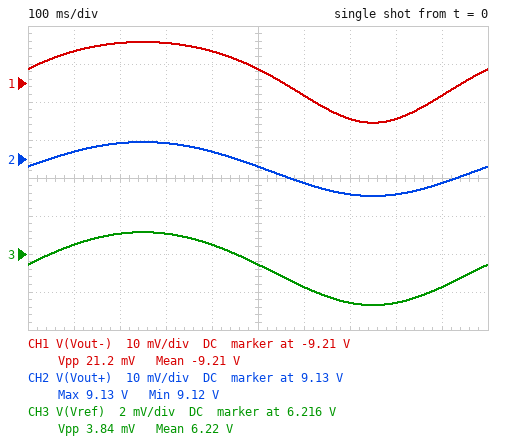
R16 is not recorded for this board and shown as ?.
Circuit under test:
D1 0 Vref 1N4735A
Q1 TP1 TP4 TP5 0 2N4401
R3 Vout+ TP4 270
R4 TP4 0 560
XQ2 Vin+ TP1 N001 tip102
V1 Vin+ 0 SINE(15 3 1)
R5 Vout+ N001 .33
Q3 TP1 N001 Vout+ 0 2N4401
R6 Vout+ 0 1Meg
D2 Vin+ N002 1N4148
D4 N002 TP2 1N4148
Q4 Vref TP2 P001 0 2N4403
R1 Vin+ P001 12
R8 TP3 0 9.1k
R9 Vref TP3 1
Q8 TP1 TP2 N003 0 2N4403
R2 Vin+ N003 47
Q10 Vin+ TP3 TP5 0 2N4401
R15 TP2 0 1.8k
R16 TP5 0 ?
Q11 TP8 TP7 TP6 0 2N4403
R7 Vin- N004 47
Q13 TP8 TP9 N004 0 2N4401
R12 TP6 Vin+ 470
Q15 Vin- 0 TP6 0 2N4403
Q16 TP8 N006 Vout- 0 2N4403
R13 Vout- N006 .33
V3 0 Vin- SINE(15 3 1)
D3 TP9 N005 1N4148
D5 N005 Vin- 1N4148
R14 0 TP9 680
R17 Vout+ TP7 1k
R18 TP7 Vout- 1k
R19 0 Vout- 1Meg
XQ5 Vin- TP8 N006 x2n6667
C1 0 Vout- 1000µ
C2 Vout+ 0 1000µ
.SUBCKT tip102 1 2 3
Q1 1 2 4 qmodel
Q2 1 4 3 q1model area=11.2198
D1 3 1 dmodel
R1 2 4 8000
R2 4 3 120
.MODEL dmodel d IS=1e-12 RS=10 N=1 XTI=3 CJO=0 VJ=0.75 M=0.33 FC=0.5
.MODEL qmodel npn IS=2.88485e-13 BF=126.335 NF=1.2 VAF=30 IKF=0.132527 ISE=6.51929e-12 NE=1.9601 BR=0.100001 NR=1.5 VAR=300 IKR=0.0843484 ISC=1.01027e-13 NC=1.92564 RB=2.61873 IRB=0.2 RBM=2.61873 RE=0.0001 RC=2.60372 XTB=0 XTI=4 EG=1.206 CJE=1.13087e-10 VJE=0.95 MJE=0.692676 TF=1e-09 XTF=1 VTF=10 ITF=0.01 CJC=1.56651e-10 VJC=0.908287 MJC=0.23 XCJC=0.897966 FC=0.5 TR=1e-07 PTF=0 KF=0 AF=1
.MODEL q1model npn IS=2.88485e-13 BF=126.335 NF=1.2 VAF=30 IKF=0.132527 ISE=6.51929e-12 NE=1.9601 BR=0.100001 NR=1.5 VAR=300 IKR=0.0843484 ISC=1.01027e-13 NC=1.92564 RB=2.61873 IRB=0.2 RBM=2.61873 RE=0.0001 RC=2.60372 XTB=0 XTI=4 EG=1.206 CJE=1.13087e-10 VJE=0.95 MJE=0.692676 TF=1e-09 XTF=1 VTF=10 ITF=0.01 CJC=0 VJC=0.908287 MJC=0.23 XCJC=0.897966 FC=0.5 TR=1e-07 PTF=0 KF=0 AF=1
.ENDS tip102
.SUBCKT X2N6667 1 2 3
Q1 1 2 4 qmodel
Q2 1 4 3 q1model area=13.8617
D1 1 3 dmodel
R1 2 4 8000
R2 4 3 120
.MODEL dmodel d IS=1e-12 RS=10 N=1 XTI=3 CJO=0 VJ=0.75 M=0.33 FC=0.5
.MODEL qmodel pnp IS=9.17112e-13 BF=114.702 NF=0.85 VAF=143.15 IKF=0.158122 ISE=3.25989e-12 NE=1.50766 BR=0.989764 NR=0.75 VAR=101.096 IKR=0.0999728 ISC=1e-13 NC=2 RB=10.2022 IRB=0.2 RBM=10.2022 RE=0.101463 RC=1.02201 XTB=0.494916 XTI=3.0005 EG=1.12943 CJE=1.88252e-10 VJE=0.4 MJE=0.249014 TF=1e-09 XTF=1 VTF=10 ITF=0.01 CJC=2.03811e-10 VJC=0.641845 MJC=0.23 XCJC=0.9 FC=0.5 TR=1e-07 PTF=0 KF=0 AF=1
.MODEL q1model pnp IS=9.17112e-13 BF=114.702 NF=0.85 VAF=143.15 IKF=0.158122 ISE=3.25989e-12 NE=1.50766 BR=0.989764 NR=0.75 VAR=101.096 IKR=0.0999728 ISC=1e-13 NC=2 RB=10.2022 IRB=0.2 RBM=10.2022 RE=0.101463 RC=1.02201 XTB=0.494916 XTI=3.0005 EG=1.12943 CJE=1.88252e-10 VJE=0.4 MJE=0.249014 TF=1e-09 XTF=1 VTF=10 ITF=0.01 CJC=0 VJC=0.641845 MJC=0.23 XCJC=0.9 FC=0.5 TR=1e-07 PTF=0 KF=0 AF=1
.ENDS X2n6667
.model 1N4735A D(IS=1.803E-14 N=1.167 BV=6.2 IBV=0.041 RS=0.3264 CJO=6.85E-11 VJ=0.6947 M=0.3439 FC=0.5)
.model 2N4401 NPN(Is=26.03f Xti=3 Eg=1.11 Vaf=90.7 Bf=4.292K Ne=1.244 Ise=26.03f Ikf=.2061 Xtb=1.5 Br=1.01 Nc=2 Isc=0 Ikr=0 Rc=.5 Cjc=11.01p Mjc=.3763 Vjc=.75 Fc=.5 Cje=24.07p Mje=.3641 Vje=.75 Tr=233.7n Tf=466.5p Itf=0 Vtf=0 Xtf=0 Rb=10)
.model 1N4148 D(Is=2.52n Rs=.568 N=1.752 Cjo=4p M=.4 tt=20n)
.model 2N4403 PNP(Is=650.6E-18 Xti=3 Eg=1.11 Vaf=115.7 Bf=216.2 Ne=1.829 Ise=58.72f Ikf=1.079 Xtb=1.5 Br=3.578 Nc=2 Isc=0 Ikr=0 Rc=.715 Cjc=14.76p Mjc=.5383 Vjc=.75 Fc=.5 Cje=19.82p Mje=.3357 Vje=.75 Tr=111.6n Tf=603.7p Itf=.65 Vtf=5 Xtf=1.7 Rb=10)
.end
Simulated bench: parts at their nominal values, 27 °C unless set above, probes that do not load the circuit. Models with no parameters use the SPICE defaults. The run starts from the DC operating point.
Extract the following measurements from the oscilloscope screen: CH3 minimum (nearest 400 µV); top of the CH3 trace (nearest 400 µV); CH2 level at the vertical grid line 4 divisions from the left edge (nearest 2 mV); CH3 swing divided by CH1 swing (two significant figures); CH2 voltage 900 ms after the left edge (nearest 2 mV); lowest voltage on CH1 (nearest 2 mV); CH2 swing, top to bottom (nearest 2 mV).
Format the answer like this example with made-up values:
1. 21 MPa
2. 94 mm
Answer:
1. 6.2132 V
2. 6.2172 V
3. 9.132 V
4. 0.18
5. 9.124 V
6. -9.220 V
7. 14 mV
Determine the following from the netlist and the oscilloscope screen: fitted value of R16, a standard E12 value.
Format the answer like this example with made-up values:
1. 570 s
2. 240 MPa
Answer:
1. 47 Ω
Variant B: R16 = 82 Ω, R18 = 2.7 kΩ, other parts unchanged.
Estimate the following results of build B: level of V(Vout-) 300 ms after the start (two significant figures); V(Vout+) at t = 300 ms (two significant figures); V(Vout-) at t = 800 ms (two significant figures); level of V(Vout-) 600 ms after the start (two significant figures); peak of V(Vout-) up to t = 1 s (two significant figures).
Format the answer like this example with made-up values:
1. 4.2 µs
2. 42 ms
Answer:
1. -16 V
2. 9.2 V
3. -12 V
4. -14 V
5. -11 V
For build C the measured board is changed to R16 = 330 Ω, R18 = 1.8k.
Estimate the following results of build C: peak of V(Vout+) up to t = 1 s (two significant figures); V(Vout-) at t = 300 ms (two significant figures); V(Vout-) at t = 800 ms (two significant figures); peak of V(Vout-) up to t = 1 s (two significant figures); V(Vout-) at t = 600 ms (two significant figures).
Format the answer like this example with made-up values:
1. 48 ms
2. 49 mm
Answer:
1. 9.3 V
2. -16 V
3. -12 V
4. -11 V
5. -14 V
